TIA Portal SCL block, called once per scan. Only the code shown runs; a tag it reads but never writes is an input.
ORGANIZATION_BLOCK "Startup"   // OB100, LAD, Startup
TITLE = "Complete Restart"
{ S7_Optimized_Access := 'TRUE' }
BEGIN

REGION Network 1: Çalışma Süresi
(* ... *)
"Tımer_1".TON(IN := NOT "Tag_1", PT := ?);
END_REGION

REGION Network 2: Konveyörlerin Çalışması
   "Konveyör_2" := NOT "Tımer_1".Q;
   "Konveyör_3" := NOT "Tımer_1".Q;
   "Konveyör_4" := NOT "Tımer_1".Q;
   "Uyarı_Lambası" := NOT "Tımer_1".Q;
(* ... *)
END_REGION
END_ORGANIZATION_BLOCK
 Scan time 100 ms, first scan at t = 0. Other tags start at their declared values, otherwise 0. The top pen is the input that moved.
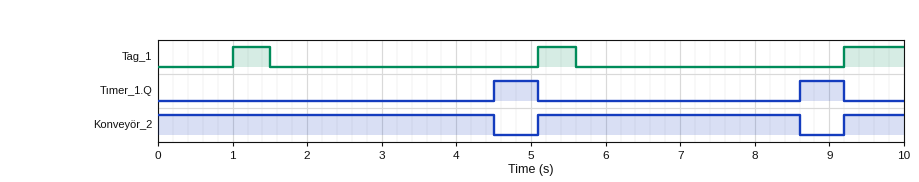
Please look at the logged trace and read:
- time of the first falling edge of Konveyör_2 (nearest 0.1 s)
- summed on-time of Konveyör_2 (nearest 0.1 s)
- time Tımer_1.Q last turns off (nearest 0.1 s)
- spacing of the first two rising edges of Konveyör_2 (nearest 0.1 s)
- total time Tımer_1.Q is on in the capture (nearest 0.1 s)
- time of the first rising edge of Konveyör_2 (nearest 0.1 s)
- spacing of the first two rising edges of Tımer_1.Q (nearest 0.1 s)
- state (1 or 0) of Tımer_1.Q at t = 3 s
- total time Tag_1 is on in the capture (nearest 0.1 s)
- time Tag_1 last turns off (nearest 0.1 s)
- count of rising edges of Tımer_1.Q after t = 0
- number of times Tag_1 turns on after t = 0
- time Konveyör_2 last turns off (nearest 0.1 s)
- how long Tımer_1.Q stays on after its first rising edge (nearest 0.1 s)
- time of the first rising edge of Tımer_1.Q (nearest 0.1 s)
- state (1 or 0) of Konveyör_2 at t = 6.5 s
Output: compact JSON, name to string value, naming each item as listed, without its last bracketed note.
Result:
{"time of the first falling edge of Konveyör_2": "4.5 s", "summed on-time of Konveyör_2": "8.8 s", "time Tımer_1.Q last turns off": "9.2 s", "spacing of the first two rising edges of Konveyör_2": "4.1 s", "total time Tımer_1.Q is on in the capture": "1.2 s", "time of the first rising edge of Konveyör_2": "5.1 s", "spacing of the first two rising edges of Tımer_1.Q": "4.1 s", "state (1 or 0) of Tımer_1.Q at t = 3 s": "0", "total time Tag_1 is on in the capture": "1.8 s", "time Tag_1 last turns off": "5.6 s", "count of rising edges of Tımer_1.Q after t = 0": "2", "number of times Tag_1 turns on after t = 0": "3", "time Konveyör_2 last turns off": "8.6 s", "how long Tımer_1.Q stays on after its first rising edge": "0.6 s", "time of the first rising edge of Tımer_1.Q": "4.5 s", "state (1 or 0) of Konveyör_2 at t = 6.5 s": "1"}
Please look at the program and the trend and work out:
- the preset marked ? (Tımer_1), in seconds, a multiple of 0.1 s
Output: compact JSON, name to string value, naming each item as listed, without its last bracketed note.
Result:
{"the preset marked ? (Tımer_1), in seconds, a multiple of 0.1 s": "3.0 s"}
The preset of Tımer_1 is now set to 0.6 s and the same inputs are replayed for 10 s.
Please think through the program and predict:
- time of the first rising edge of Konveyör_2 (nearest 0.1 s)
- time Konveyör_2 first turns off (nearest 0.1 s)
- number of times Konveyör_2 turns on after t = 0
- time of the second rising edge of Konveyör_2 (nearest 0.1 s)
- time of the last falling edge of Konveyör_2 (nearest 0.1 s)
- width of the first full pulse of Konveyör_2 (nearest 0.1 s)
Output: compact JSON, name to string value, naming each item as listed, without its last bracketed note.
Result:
{"time of the first rising edge of Konveyör_2": "1.0 s", "time Konveyör_2 first turns off": "0.6 s", "number of times Konveyör_2 turns on after t = 0": "3", "time of the second rising edge of Konveyör_2": "5.1 s", "time of the last falling edge of Konveyör_2": "6.2 s", "width of the first full pulse of Konveyör_2": "1.1 s"}
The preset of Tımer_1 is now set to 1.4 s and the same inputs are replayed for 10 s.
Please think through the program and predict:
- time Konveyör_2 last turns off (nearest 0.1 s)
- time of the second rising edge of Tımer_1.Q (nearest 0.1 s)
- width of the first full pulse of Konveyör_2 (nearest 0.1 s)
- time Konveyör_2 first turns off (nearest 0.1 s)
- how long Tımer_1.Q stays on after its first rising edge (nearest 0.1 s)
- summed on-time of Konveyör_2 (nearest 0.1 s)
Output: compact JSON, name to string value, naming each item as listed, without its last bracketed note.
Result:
{"time Konveyör_2 last turns off": "7.0 s", "time of the second rising edge of Tımer_1.Q": "7.0 s", "width of the first full pulse of Konveyör_2": "1.9 s", "time Konveyör_2 first turns off": "2.9 s", "how long Tımer_1.Q stays on after its first rising edge": "2.2 s", "summed on-time of Konveyör_2": "5.6 s"}
